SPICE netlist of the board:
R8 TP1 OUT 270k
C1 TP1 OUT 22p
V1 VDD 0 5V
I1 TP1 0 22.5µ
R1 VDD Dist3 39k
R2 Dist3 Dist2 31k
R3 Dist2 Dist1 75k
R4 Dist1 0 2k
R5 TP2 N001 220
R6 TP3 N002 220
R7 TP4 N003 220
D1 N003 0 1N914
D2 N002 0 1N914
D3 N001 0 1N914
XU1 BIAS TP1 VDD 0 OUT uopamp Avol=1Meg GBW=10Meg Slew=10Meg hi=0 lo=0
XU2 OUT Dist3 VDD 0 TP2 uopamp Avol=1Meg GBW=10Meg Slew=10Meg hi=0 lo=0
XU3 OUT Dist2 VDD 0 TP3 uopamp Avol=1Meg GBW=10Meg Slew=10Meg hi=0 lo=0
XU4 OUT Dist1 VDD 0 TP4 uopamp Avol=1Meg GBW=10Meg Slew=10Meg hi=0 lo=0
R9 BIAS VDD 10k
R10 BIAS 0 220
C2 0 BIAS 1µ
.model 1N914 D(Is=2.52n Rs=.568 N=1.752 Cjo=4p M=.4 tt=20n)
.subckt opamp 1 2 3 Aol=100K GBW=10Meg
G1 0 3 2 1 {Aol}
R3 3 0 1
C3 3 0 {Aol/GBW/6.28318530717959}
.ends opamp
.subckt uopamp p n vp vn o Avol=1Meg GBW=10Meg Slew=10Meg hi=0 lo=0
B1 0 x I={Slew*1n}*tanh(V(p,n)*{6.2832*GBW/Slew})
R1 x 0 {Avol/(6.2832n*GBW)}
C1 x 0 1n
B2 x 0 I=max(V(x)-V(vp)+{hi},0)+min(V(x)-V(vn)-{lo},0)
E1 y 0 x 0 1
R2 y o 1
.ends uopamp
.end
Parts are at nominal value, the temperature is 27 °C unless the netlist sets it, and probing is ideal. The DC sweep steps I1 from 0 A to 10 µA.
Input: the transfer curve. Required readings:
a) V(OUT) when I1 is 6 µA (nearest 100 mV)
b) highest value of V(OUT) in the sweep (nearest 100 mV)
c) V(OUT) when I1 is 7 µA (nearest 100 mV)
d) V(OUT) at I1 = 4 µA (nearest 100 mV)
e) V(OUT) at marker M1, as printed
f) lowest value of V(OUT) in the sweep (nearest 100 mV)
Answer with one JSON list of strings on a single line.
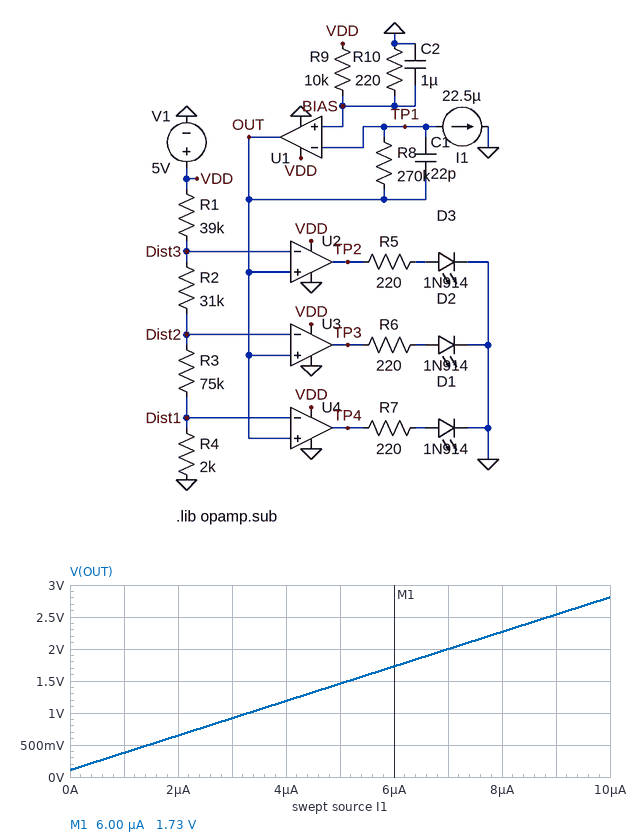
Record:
["1.7 V", "2.8 V", "2.0 V", "1.2 V", "1.73 V", "100 mV"]
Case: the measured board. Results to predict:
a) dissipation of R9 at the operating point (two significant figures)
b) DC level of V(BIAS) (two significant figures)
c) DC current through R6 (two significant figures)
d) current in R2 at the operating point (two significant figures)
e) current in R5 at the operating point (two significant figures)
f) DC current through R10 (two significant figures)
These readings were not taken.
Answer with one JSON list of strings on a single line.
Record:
["2.4 mW", "110 mV", "19 mA", "34 µA", "19 mA", "490 µA"]
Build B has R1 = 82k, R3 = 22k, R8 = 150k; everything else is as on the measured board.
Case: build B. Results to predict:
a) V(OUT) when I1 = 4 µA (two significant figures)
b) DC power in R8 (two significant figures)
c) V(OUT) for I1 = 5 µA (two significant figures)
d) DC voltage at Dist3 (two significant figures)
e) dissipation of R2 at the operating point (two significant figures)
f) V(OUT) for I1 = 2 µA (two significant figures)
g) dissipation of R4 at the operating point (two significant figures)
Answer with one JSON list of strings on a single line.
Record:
["710 mV", "76 µW", "860 mV", "2.0 V", "41 µW", "410 mV", "2.7 µW"]
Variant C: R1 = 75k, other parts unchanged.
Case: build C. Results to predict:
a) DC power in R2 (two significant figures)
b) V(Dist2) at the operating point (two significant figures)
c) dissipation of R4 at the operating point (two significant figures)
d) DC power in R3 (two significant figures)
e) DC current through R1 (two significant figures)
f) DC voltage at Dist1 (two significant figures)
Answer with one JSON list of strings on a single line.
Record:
["23 µW", "2.1 V", "1.5 µW", "56 µW", "27 µA", "55 mV"]
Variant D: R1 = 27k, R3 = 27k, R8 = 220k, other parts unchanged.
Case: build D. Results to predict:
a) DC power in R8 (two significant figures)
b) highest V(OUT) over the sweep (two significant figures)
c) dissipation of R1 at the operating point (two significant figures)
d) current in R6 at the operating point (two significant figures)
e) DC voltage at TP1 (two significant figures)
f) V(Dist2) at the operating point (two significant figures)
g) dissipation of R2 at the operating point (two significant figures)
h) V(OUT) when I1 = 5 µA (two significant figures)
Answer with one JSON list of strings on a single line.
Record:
["110 µW", "2.3 V", "89 µW", "19 mA", "53 mV", "1.7 V", "100 µW", "1.2 V"]
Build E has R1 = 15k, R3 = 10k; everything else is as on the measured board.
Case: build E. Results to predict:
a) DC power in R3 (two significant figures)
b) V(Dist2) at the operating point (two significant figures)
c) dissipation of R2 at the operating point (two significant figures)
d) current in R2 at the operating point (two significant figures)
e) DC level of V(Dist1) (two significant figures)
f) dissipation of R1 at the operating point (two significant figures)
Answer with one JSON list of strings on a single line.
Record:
["74 µW", "1.0 V", "230 µW", "86 µA", "170 mV", "110 µW"]
